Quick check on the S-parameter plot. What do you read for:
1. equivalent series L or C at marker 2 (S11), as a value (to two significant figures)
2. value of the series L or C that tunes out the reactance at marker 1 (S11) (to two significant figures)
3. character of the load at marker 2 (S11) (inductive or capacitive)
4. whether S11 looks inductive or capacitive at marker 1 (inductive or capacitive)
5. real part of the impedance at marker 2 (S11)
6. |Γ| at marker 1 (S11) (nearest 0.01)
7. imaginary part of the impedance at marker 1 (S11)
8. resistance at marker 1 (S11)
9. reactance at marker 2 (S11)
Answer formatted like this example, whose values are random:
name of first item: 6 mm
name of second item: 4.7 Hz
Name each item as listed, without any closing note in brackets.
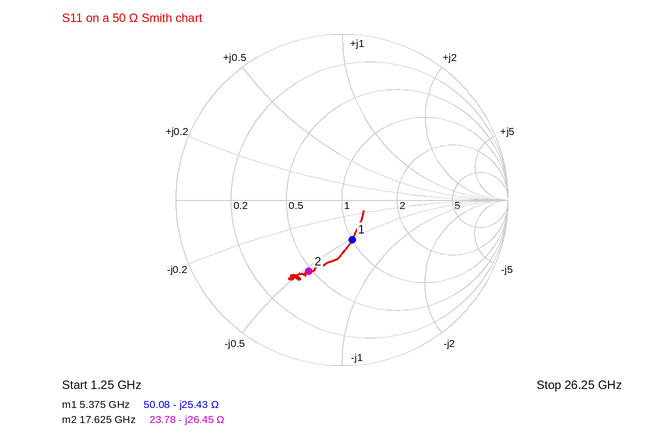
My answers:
equivalent series L or C at marker 2 (S11), as a value: 340 fF
value of the series L or C that tunes out the reactance at marker 1 (S11): 750 pH
character of the load at marker 2 (S11): capacitive
whether S11 looks inductive or capacitive at marker 1: capacitive
real part of the impedance at marker 2: 23.78 Ω
|Γ| at marker 1 (S11): 0.25
imaginary part of the impedance at marker 1: -25.43 Ω
resistance at marker 1: 50.08 Ω
reactance at marker 2: -26.45 Ω
